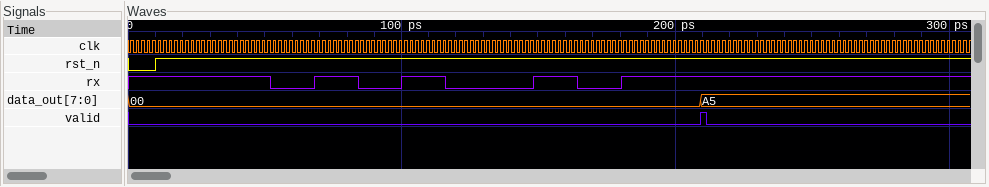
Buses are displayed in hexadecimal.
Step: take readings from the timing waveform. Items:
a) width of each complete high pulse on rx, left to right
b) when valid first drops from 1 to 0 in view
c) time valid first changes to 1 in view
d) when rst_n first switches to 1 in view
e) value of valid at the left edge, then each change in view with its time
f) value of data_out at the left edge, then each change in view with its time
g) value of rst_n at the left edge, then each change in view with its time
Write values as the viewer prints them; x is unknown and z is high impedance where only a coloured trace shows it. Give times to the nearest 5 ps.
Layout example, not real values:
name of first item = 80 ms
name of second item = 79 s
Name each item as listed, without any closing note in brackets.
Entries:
width of each complete high pulse on rx, left to right = 15 ps, 15 ps, 15 ps
when valid first drops from 1 to 0 in view = 210 ps
time valid first changes to 1 in view = 210 ps
when rst_n first switches to 1 in view = 10 ps
value of valid at the left edge, then each change in view with its time = 0, 1 at 210 ps, 0 at 210 ps
value of data_out at the left edge, then each change in view with its time = 00, A5 at 210 ps
value of rst_n at the left edge, then each change in view with its time = 0, 1 at 10 ps
